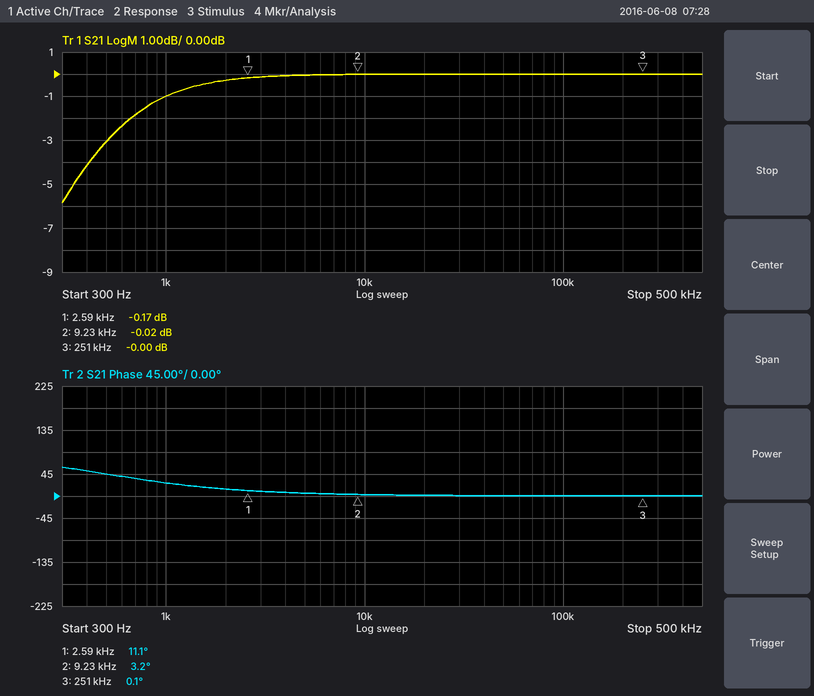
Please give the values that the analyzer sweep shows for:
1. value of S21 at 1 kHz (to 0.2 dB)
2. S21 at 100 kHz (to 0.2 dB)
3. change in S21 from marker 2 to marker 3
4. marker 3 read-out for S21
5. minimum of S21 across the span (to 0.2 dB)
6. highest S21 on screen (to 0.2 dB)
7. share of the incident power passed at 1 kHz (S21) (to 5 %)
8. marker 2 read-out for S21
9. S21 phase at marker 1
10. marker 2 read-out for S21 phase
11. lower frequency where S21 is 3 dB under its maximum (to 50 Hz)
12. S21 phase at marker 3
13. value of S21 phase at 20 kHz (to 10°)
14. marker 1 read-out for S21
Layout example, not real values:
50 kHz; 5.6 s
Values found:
-1.0 dB; 0.0 dB; 0.02 dB; -0.00 dB; -5.8 dB; 0.0 dB; 80 %; -0.02 dB; 11.1°; 3.2°; 500 Hz; 0.1°; 0°; -0.17 dB
